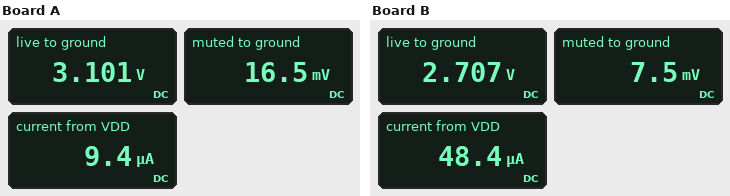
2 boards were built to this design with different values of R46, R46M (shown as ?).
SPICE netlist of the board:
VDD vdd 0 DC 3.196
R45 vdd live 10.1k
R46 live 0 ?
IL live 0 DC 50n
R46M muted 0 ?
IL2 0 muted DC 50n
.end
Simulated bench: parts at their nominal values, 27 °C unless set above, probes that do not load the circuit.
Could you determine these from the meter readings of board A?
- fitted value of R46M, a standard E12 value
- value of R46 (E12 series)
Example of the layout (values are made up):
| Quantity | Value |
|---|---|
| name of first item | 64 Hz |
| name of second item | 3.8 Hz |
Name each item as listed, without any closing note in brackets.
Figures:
| Quantity | Value |
|---|---|
| fitted value of R46M, a standard E12 value | 330 kΩ |
| value of R46 | 330 kΩ |
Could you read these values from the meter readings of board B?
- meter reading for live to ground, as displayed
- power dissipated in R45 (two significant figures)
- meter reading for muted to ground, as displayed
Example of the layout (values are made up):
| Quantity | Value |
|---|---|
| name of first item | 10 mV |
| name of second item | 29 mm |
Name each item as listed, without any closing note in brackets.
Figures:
| Quantity | Value |
|---|---|
| meter reading for live to ground, as displayed | 2.707 V |
| power dissipated in R45 | 24 µW |
| meter reading for muted to ground, as displayed | 7.5 mV |
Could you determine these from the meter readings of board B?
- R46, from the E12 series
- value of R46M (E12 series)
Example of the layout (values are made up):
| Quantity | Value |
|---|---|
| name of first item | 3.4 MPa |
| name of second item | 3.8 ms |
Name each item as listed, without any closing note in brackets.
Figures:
| Quantity | Value |
|---|---|
| R46, from the E12 series | 56 kΩ |
| value of R46M | 150 kΩ |
